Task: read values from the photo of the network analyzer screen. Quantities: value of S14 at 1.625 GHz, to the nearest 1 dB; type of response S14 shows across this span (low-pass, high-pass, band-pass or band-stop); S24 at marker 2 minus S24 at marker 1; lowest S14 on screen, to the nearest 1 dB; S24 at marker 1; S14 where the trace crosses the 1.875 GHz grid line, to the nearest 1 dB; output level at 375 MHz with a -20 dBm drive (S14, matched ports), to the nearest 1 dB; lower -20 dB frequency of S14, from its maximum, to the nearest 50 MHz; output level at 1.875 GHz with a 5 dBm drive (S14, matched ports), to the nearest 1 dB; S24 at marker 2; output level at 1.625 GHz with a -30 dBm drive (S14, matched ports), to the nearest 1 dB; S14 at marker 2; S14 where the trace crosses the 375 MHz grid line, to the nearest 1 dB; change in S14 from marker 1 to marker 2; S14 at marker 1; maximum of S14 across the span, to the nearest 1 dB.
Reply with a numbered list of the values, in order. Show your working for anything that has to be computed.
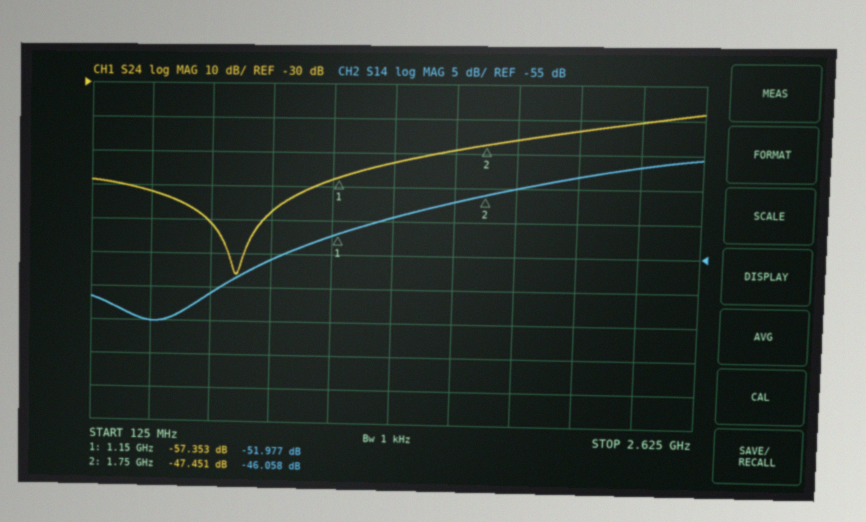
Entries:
1. -47 dB
2. high-pass
3. -47.451 − (-57.353) = 9.902 dB
4. -65 dB
5. -57.353 dB
6. -45 dB
7. -20 dBm + (-65 dB) = -85 dBm
8. 650 MHz
9. 5 dBm + (-45 dB) = -40 dBm
10. -47.451 dB
11. -30 dBm + (-47 dB) = -77 dBm
12. -46.058 dB
13. -65 dB
14. -46.058 − (-51.977) = 5.919 dB
15. -51.977 dB
16. -41 dB
